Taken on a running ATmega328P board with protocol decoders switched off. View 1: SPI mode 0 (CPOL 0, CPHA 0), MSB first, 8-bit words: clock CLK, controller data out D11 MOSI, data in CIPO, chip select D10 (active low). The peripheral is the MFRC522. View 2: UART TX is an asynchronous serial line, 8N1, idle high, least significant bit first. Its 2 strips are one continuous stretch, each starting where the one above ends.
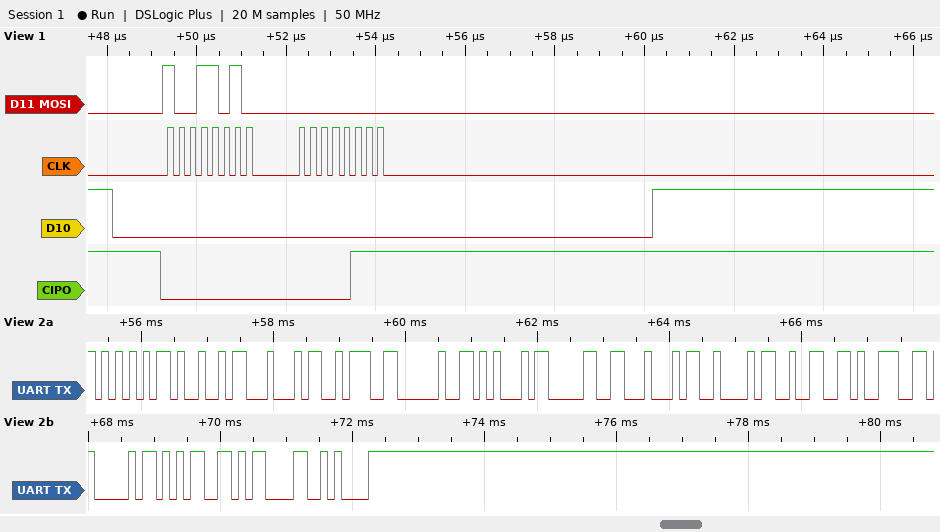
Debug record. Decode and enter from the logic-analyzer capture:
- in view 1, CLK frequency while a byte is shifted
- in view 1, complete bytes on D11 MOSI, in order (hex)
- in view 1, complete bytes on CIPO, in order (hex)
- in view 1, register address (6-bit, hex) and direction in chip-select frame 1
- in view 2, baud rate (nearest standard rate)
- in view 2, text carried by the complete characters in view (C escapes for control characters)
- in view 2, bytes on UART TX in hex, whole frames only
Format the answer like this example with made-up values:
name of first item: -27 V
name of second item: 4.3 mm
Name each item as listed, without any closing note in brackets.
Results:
in view 1, CLK frequency while a byte is shifted: 4 MHz
in view 1, complete bytes on D11 MOSI, in order: 0x9A 0x00
in view 1, complete bytes on CIPO, in order: 0x00 0x07
in view 1, register address (6-bit, hex) and direction in chip-select frame 1: 0x0D read
in view 2, baud rate: 9600 baud
in view 2, text carried by the complete characters in view: "UID: E0DB29A5\r\n"
in view 2, bytes on UART TX in hex, whole frames only: 55 49 44 3A 20 45 30 44 42 32 39 41 35 0D 0A
